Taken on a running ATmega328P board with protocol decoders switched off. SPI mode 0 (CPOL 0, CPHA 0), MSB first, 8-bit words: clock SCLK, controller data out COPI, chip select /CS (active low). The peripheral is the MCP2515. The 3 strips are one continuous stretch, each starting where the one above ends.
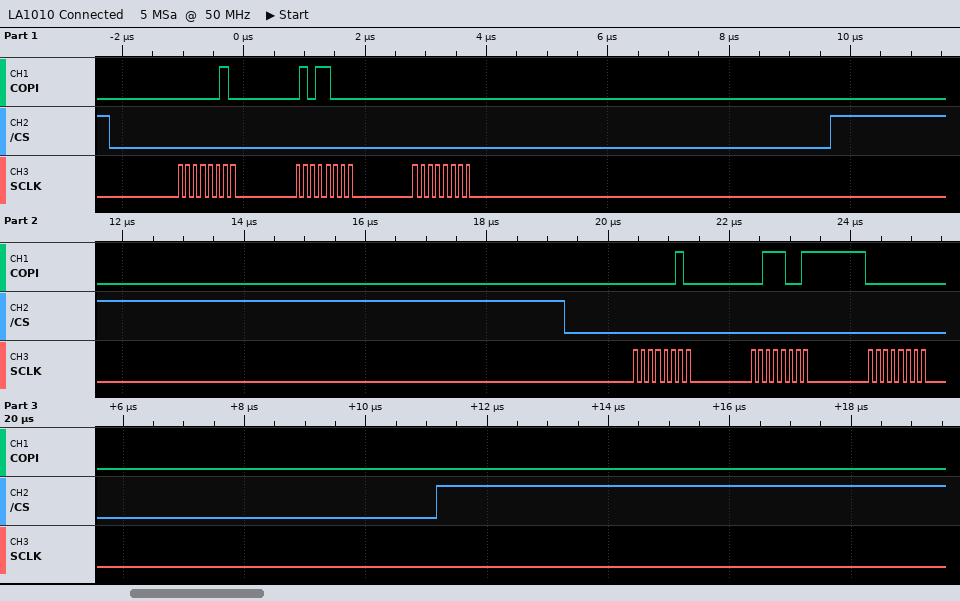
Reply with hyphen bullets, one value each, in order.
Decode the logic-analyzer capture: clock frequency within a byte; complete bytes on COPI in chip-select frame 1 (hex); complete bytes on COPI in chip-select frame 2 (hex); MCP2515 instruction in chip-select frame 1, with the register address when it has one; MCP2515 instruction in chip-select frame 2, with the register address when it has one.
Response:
- 8 MHz
- 02 58 00
- 02 39 00
- WRITE 0x58
- WRITE 0x39
